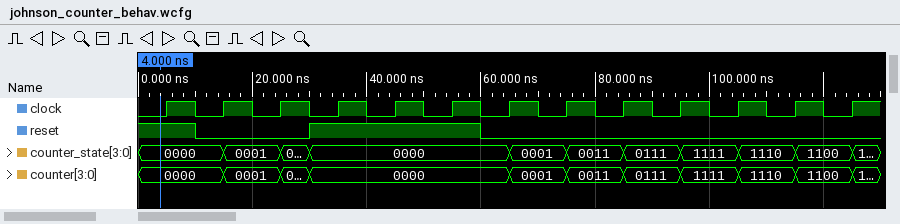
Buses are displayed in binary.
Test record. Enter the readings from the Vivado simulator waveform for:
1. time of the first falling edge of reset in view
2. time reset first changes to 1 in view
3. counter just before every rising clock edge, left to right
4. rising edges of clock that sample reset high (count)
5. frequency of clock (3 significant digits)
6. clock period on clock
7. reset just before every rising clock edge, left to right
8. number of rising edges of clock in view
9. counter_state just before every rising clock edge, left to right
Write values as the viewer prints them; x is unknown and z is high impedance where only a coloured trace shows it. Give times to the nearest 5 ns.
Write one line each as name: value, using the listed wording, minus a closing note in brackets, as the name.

time of the first falling edge of reset in view: 10 ns
time reset first changes to 1 in view: 30 ns
counter just before every rising clock edge, left to right: 0000, 0000, 0001, 0000, 0000, 0000, 0000, 0001, 0011, 0111, 1111, 1110, 1100
rising edges of clock that sample reset high: 4
frequency of clock: 100 MHz
clock period on clock: 10 ns
reset just before every rising clock edge, left to right: 1 0 0 1 1 1 0 0 0 0 0 0 0
number of rising edges of clock in view: 13
counter_state just before every rising clock edge, left to right: 0000, 0000, 0001, 0000, 0000, 0000, 0000, 0001, 0011, 0111, 1111, 1110, 1100
